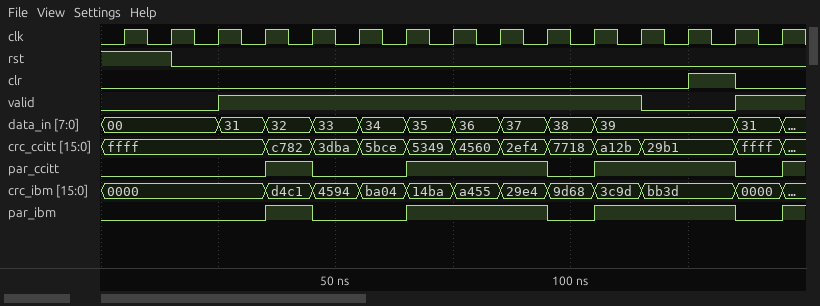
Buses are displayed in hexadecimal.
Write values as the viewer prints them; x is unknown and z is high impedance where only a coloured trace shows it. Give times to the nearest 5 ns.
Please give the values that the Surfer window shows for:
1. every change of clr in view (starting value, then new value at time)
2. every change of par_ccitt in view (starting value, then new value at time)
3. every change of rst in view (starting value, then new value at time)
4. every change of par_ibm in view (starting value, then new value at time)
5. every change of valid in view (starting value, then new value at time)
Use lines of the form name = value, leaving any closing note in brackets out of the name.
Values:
every change of clr in view = 0, 1 at 125 ns, 0 at 135 ns
every change of par_ccitt in view = 0, 1 at 35 ns, 0 at 45 ns, 1 at 65 ns, 0 at 95 ns, 1 at 105 ns, 0 at 135 ns, 1 at 145 ns
every change of rst in view = 1, 0 at 15 ns
every change of par_ibm in view = 0, 1 at 35 ns, 0 at 45 ns, 1 at 65 ns, 0 at 95 ns, 1 at 105 ns, 0 at 135 ns, 1 at 145 ns
every change of valid in view = 0, 1 at 25 ns, 0 at 115 ns, 1 at 135 ns
